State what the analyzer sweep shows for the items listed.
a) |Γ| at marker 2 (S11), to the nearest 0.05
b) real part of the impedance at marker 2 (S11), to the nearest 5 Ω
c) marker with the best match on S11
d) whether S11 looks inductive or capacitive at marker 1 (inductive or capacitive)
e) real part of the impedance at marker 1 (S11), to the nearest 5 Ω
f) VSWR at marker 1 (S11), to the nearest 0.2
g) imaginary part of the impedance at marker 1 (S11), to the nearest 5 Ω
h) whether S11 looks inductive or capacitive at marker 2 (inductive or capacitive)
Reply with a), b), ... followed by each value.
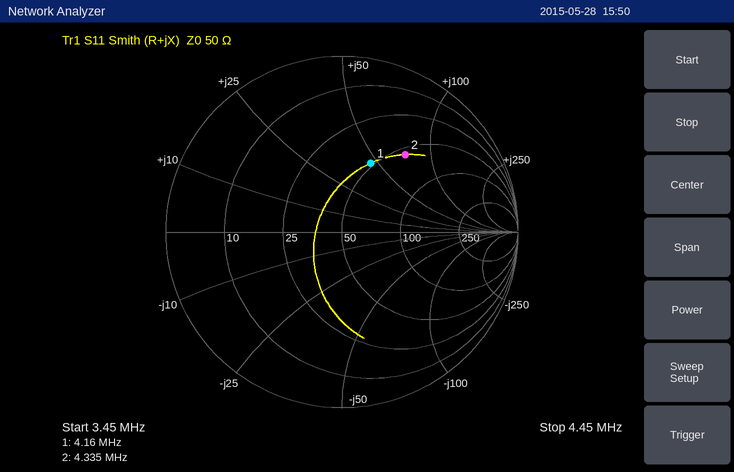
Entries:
a) 0.55
b) 55 Ω
c) marker 1
d) inductive
e) 50 Ω
f) 2.4
g) +45 Ω
h) inductive
